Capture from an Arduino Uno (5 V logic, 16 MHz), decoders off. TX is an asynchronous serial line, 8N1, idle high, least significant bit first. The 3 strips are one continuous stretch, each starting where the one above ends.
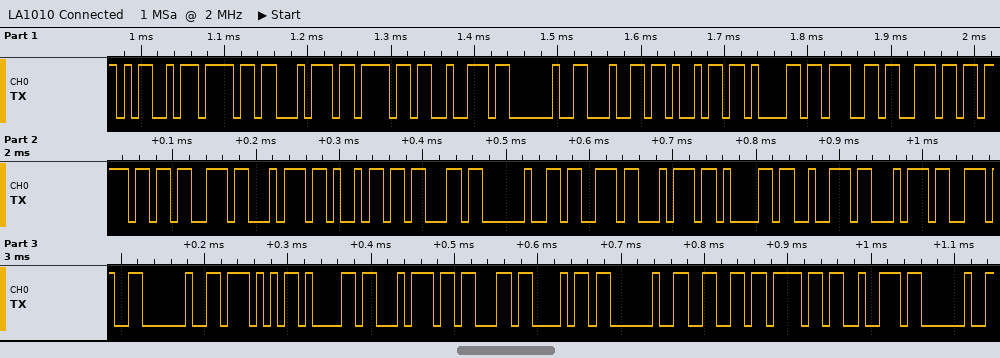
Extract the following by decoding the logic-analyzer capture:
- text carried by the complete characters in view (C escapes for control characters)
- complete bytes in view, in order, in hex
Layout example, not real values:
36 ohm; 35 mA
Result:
"Motor diagnostic start. Watch for "; 4D 6F 74 6F 72 20 64 69 61 67 6E 6F 73 74 69 63 20 73 74 61 72 74 2E 20 57 61 74 63 68 20 66 6F 72 20
